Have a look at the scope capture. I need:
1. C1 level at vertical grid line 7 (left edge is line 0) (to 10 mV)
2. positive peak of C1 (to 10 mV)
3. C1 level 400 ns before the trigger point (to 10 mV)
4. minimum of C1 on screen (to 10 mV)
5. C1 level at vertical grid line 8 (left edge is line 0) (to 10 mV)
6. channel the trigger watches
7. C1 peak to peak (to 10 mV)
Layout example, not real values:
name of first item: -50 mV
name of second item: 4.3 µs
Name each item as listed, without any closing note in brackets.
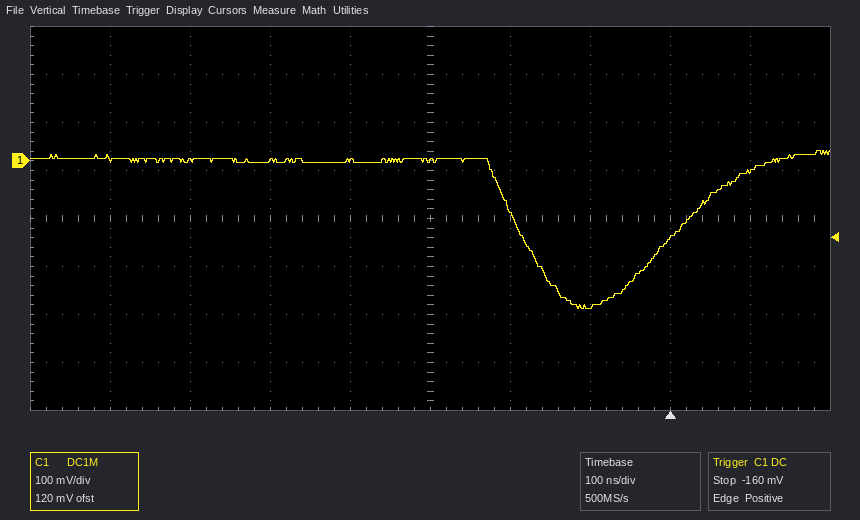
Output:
C1 level at vertical grid line 7 (left edge is line 0): -300 mV
positive peak of C1: 20 mV
C1 level 400 ns before the trigger point: 0 mV
minimum of C1 on screen: -310 mV
C1 level at vertical grid line 8 (left edge is line 0): -160 mV
channel the trigger watches: C1
C1 peak to peak: 330 mV
